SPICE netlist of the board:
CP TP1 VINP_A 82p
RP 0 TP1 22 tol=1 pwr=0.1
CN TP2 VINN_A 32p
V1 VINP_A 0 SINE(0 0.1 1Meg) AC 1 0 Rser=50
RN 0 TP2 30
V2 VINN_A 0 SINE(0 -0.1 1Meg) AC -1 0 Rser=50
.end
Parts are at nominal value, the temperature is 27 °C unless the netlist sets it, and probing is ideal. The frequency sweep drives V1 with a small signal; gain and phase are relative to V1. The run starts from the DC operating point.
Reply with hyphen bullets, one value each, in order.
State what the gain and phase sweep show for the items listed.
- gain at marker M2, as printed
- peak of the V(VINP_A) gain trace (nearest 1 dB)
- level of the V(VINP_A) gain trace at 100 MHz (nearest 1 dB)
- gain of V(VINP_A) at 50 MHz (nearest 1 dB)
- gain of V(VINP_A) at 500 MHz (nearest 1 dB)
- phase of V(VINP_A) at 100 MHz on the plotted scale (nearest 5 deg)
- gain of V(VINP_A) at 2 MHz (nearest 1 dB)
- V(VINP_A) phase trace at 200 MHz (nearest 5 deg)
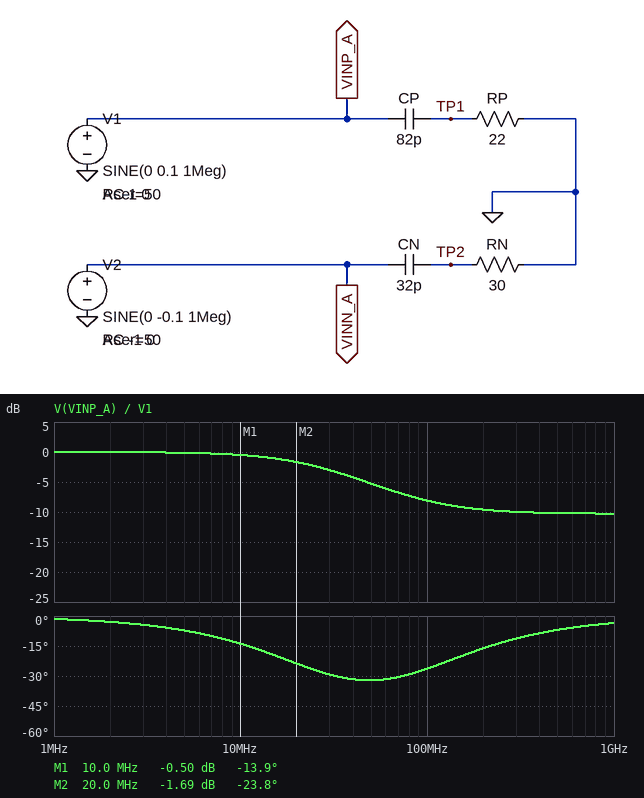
- -1.69 dB
- 0 dB
- -8 dB
- -5 dB
- -10 dB
- -25 deg
- 0 dB
- -15 deg
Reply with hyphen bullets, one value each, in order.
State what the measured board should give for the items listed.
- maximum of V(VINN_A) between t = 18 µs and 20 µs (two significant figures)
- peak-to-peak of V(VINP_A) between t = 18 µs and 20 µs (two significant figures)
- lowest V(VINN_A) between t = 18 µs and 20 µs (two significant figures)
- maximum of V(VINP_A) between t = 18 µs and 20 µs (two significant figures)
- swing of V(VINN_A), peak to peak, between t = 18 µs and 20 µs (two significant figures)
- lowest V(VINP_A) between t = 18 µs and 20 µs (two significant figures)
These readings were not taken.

- 100 mV
- 200 mV
- -100 mV
- 100 mV
- 200 mV
- -100 mV
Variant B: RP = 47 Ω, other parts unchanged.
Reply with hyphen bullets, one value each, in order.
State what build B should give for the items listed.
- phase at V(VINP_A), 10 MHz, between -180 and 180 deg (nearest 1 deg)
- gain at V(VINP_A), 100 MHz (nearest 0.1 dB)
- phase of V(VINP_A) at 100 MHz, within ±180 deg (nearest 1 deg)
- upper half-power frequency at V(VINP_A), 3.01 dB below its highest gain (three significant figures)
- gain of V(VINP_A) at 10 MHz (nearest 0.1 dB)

- -13 deg
- -5.8 dB
- -11 deg
- 27.5 MHz
- -0.7 dB
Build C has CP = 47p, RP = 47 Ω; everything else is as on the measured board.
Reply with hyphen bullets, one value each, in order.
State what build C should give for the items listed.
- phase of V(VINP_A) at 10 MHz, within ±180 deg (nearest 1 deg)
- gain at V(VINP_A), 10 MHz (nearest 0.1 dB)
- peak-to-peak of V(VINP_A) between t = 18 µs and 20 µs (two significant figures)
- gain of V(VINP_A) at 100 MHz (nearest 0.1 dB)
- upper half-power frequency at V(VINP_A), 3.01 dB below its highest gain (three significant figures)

- -8 deg
- -0.3 dB
- 200 mV
- -5.0 dB
- 47.9 MHz
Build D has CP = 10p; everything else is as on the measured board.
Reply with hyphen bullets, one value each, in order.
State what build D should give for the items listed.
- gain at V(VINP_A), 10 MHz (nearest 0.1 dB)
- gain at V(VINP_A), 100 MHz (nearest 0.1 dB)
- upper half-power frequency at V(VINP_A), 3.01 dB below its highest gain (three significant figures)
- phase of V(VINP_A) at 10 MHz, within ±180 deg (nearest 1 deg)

- 0 dB
- -0.7 dB
- 245 MHz
- -2 deg
